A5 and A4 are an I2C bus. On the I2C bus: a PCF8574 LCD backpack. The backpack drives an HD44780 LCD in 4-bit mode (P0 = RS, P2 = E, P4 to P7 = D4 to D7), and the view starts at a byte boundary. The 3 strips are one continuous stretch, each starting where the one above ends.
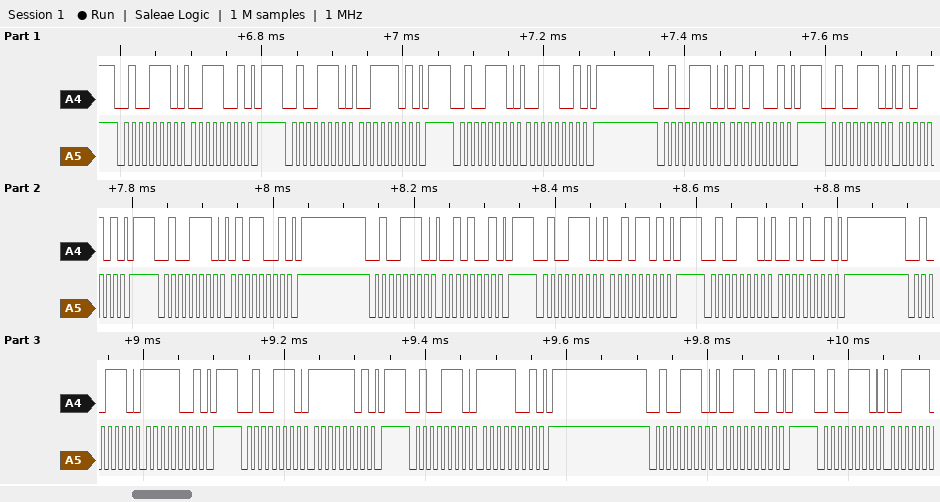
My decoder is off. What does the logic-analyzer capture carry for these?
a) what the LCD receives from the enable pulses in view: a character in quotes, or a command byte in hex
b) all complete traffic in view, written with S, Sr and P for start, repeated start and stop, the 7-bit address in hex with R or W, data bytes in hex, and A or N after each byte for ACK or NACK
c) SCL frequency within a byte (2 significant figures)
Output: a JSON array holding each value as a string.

["'5' '/'", "S 27W A 39 A P S 27W A 3D A P S 27W A 39 A P S 27W A 59 A P S 27W A 5D A P S 27W A 59 A P S 27W A 29 A P S 27W A 2D A P S 27W A 29 A P S 27W A F9 A P S 27W A FD A P S 27W A F9 A P S 27W A 39 A P S 27W A", "100 kHz"]
